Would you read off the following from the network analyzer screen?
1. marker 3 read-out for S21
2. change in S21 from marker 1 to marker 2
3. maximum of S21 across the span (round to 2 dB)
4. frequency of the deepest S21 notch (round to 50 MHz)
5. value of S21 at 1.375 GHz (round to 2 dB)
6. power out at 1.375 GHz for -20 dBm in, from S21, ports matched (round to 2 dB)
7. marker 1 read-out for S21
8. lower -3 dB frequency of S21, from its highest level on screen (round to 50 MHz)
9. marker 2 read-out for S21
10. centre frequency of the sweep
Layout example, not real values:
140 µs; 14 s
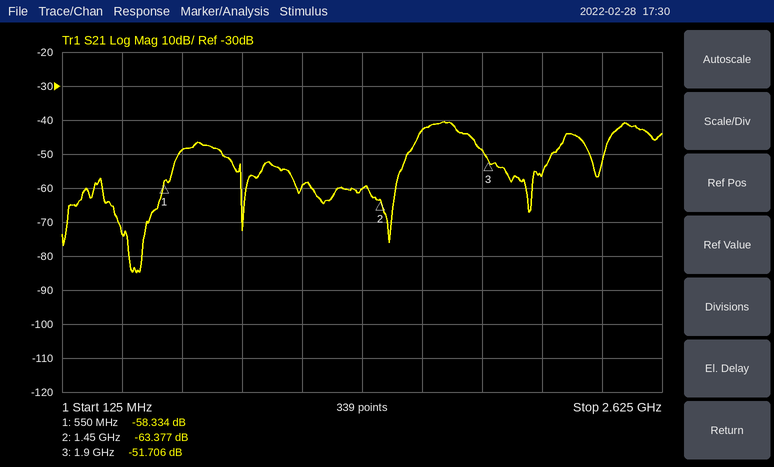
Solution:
-51.706 dB; -5.043 dB; -40 dB; 450 MHz; -60 dB; -80 dBm; -58.334 dB; 1.60 GHz; -63.377 dB; 1.375 GHz
